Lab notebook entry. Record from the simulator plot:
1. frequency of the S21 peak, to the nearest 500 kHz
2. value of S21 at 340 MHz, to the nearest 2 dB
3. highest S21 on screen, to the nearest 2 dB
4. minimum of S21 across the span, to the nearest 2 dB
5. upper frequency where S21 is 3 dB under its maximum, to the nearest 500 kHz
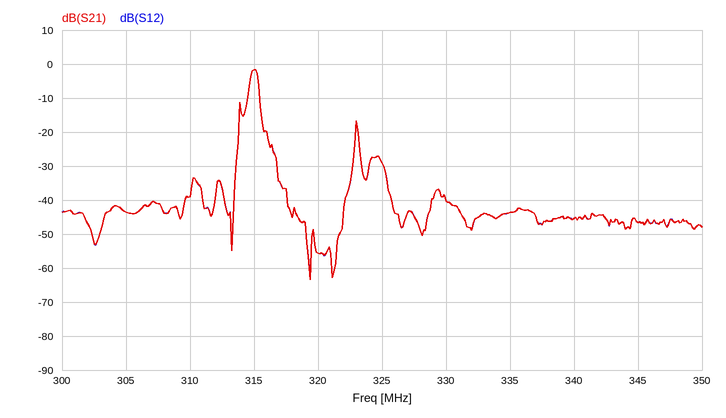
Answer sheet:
315.0 MHz
-46 dB
-2 dB
-64 dB
315.5 MHz
